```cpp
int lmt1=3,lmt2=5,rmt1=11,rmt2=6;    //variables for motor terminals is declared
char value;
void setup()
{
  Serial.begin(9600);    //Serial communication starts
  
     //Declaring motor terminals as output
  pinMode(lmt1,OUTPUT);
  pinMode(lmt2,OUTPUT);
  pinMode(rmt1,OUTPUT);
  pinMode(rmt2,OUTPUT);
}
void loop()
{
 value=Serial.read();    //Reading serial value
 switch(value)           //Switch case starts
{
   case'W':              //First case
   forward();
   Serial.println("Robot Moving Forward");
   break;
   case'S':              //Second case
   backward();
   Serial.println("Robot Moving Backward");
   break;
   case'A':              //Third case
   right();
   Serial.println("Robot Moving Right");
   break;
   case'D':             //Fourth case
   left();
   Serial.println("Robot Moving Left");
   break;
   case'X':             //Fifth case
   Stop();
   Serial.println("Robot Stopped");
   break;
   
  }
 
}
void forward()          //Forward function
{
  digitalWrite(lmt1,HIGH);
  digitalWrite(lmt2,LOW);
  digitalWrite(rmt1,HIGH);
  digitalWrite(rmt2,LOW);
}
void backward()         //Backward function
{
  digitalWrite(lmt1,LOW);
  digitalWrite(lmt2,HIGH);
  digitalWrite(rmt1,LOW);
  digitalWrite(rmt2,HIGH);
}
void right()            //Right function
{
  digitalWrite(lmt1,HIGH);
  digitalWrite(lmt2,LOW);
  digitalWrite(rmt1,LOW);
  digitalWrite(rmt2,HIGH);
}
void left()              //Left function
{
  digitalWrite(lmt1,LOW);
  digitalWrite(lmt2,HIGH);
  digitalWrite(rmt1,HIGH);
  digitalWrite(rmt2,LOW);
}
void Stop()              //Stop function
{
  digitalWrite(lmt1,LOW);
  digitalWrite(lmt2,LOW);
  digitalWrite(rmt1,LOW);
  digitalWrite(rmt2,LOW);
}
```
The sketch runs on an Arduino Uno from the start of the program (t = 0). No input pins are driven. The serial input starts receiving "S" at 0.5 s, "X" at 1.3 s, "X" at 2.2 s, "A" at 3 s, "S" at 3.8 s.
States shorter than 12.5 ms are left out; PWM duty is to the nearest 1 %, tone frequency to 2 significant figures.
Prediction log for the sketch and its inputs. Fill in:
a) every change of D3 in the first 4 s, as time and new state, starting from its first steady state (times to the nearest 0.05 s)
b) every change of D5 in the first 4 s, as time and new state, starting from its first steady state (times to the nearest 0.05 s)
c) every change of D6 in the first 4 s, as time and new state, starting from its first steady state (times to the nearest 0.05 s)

0 s low; 3 s high; 3.8 s low
0 s low; 0.5 s high; 1.3 s low; 3.8 s high
0 s low; 0.5 s high; 1.3 s low; 3 s high
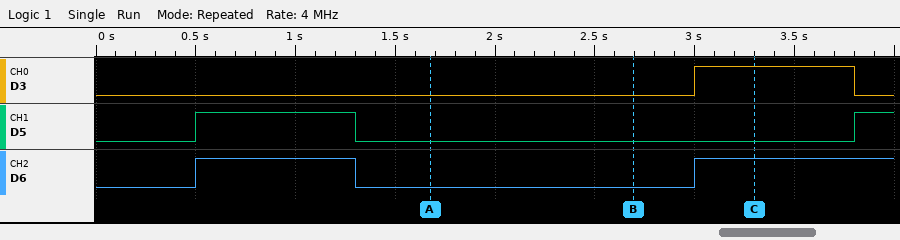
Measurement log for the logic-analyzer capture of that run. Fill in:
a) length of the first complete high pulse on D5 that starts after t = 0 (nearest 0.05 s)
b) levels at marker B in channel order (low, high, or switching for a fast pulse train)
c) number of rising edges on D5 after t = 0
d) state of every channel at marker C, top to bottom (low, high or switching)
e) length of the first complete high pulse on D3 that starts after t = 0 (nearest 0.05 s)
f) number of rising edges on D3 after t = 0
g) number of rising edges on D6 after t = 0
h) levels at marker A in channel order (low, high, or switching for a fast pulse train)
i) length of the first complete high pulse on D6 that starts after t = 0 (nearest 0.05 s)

0.80 s
D3 low, D5 low, D6 low
2
D3 high, D5 low, D6 high
0.80 s
1
2
D3 low, D5 low, D6 low
0.80 s
